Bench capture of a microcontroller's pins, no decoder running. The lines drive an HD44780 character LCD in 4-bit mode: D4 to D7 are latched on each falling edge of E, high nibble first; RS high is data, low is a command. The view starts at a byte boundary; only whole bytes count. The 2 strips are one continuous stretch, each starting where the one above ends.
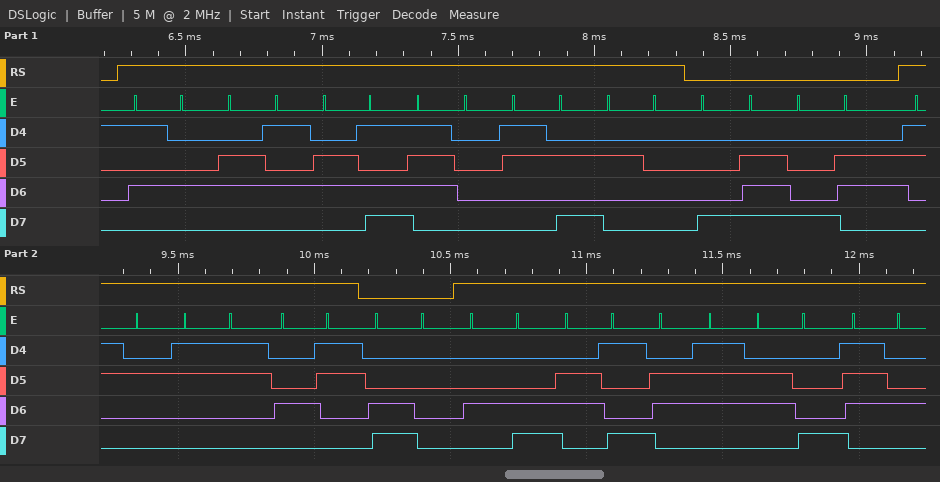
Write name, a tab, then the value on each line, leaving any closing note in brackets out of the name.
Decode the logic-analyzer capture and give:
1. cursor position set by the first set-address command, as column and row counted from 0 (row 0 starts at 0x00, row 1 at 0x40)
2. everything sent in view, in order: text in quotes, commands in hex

cursor position set by the first set-address command, as column and row counted from 0	column 14, row 0
everything sent in view, in order: text in quotes, commands in hex	"Temp: " 0x8E 0x86 "23C" 0xC0 "Light"
